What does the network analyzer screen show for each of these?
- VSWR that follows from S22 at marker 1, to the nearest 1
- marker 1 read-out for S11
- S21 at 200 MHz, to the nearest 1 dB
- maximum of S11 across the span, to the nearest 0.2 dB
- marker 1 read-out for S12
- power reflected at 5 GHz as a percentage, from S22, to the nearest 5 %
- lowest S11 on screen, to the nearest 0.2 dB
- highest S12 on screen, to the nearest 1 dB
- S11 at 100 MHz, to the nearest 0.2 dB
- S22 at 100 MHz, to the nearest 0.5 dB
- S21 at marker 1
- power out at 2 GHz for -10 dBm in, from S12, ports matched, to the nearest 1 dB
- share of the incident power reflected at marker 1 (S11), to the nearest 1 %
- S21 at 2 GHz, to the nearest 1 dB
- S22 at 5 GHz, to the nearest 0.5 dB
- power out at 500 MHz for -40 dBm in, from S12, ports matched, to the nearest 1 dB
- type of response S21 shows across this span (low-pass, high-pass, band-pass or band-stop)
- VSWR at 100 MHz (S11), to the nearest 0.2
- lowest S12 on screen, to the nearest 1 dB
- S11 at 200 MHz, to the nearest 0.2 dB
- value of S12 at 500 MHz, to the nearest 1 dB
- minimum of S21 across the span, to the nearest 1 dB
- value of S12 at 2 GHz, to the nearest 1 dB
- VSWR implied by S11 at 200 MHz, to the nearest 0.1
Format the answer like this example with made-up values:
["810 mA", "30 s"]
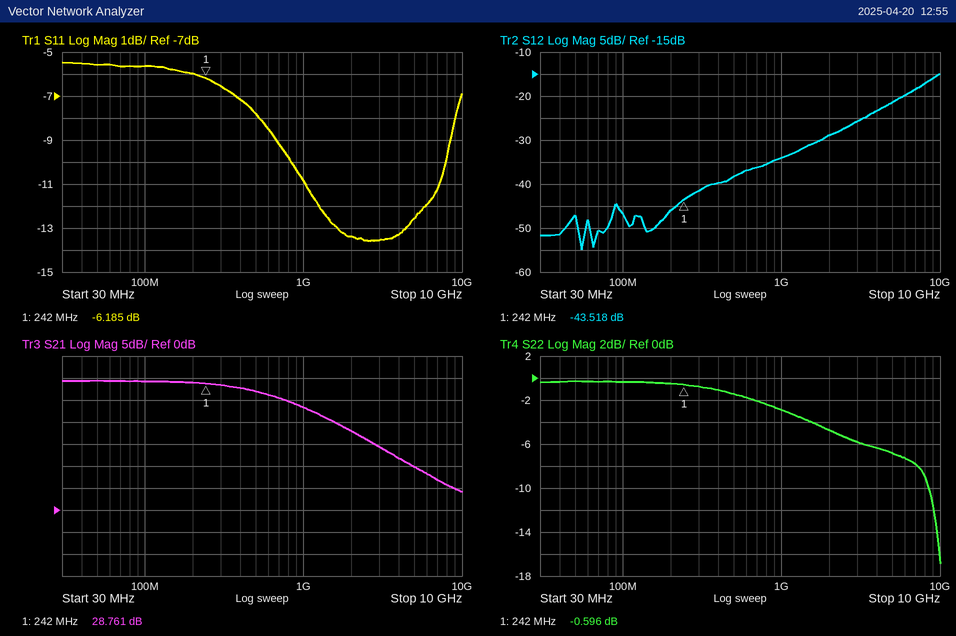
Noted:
["29", "-6.185 dB", "29 dB", "-5.4 dB", "-43.518 dB", "20 %", "-13.6 dB", "-15 dB", "-5.6 dB", "-0.5 dB", "28.761 dB", "-39 dBm", "24 %", "18 dB", "-7.0 dB", "-78 dBm", "low-pass", "3.2", "-55 dB", "-6.0 dB", "-38 dB", "4 dB", "-29 dB", "3.0"]
